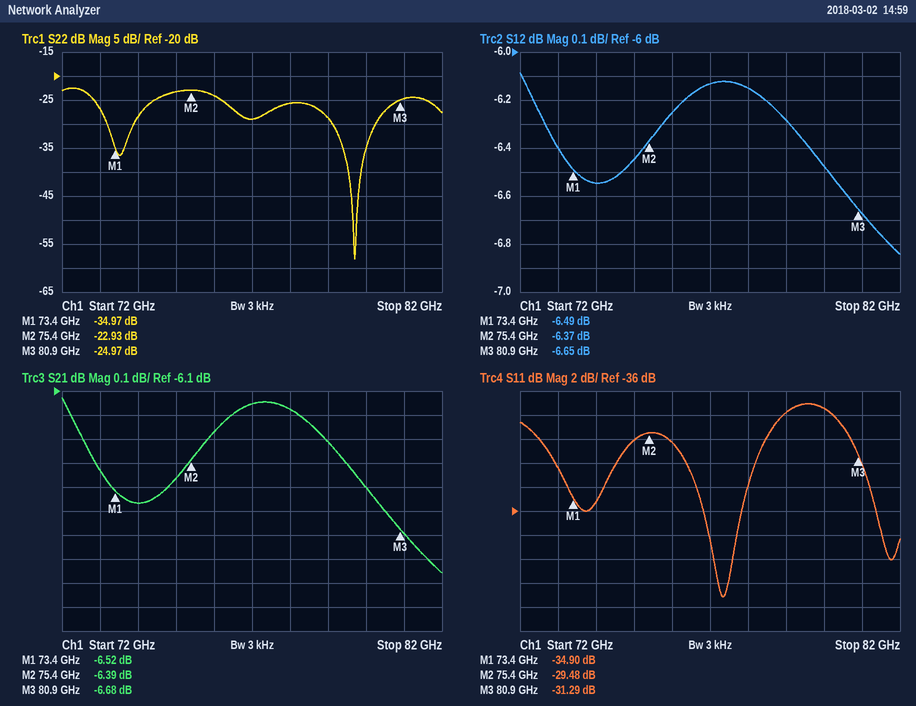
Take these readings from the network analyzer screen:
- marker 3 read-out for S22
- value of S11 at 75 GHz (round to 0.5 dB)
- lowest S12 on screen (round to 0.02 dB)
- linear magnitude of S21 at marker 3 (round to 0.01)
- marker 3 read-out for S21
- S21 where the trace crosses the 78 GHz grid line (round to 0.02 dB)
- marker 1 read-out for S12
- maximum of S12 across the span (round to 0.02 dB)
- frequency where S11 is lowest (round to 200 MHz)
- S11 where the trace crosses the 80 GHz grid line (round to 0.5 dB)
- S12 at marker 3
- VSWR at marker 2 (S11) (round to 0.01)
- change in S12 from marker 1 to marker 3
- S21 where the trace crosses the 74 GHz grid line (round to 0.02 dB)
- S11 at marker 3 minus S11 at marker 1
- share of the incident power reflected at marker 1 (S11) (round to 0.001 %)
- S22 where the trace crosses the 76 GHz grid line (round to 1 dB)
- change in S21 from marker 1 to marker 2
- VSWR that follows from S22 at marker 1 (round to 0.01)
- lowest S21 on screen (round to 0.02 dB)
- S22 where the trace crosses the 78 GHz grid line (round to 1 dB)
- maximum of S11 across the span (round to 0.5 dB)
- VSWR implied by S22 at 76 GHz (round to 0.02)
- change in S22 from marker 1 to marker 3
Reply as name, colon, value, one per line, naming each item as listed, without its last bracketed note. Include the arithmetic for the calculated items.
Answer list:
marker 3 read-out for S22: -24.97 dB
value of S11 at 75 GHz: -30.0 dB
lowest S12 on screen: -6.84 dB
linear magnitude of S21 at marker 3: 10^(-6.68/20) ≈ 0.46
marker 3 read-out for S21: -6.68 dB
S21 where the trace crosses the 78 GHz grid line: -6.18 dB
marker 1 read-out for S12: -6.49 dB
maximum of S12 across the span: -6.08 dB
frequency where S11 is lowest: 77.4 GHz
S11 where the trace crosses the 80 GHz grid line: -27.5 dB
S12 at marker 3: -6.65 dB
VSWR at marker 2 (S11): (1 + 0.0336)/(1 − 0.0336) ≈ 1.07
change in S12 from marker 1 to marker 3: -6.65 − (-6.49) = -0.16 dB
S21 where the trace crosses the 74 GHz grid line: -6.56 dB
S11 at marker 3 minus S11 at marker 1: -31.29 − (-34.9) = 3.61 dB
share of the incident power reflected at marker 1 (S11): 10^(-34.9/10) ≈ 0.032 %
S22 where the trace crosses the 76 GHz grid line: -24 dB
change in S21 from marker 1 to marker 2: -6.39 − (-6.52) = 0.13 dB
VSWR that follows from S22 at marker 1: (1 + 0.0178)/(1 − 0.0178) ≈ 1.04
lowest S21 on screen: -6.86 dB
S22 where the trace crosses the 78 GHz grid line: -26 dB
maximum of S11 across the span: -27.0 dB
VSWR implied by S22 at 76 GHz: |Γ| = 10^(-24/20) = 0.0631; VSWR = (1 + 0.0631)/(1 − 0.0631) ≈ 1.13, so 1.14 to the nearest 0.02
change in S22 from marker 1 to marker 3: -24.97 − (-34.97) = 10.00 dB
